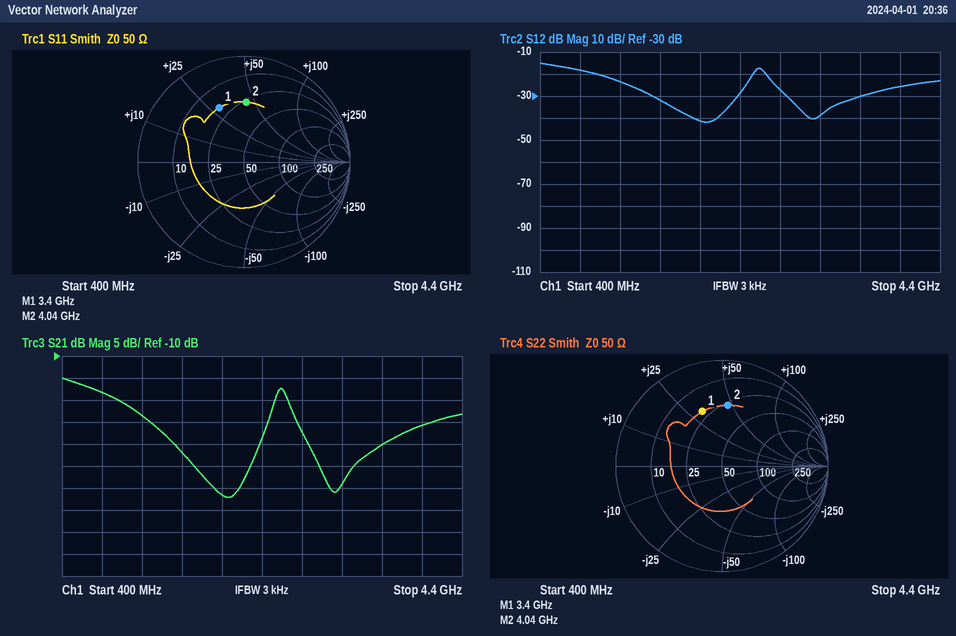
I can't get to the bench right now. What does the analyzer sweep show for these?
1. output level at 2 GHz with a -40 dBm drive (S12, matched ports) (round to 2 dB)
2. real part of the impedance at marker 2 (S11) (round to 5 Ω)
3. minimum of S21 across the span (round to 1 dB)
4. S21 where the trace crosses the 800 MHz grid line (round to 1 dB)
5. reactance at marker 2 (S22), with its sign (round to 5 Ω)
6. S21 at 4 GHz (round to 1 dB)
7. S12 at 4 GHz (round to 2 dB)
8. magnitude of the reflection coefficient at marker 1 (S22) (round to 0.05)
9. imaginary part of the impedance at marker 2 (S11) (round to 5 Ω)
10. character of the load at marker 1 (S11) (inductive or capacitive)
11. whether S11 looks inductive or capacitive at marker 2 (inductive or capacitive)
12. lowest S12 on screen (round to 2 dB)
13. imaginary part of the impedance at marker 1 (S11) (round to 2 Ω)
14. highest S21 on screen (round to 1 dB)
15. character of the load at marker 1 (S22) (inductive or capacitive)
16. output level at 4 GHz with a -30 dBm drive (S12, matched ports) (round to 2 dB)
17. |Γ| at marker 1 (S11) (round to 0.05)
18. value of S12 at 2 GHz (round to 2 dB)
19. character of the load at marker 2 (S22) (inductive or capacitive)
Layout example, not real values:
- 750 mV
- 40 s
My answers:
- -82 dBm
- 25 Ω
- -42 dB
- -18 dB
- +45 Ω
- -26 dB
- -26 dB
- 0.55
- +45 Ω
- inductive
- inductive
- -42 dB
- +28 Ω
- -15 dB
- inductive
- -56 dBm
- 0.55
- -42 dB
- inductive
